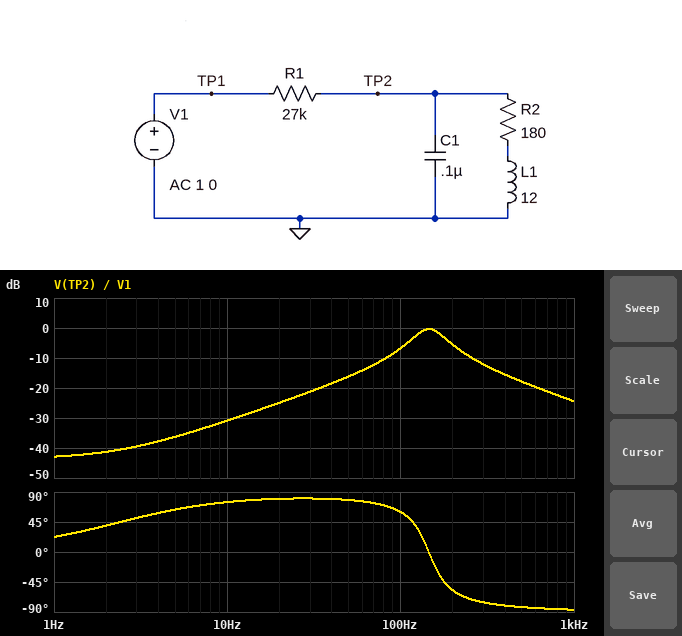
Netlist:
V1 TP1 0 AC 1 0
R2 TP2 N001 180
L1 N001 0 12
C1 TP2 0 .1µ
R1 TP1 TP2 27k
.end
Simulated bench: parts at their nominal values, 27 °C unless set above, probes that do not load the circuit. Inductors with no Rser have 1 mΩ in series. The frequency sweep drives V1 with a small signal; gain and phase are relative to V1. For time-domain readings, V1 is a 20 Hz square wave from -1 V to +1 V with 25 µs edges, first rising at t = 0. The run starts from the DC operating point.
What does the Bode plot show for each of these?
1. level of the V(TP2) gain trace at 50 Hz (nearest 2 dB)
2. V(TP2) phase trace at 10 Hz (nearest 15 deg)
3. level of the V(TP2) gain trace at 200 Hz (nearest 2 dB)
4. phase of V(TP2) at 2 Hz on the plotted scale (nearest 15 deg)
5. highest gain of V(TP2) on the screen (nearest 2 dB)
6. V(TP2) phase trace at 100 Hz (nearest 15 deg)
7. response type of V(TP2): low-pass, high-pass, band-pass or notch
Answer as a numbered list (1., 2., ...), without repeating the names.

1. -16 dB
2. 75 deg
3. -6 dB
4. 45 deg
5. 0 dB
6. 60 deg
7. band-pass
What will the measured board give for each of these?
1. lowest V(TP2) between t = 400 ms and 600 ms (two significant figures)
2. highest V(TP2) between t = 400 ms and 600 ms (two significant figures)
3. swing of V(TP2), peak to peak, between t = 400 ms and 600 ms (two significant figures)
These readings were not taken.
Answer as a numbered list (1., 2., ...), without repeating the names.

1. -610 mV
2. 610 mV
3. 1.2 V
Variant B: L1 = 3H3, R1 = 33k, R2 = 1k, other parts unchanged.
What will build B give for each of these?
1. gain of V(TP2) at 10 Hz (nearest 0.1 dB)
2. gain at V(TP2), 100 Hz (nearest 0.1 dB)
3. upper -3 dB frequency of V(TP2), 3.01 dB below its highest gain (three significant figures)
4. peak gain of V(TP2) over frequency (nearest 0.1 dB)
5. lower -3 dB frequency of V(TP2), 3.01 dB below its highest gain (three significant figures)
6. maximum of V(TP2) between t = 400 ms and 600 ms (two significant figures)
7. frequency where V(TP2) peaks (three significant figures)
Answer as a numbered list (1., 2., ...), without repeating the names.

1. -30.4 dB
2. -22.3 dB
3. 333 Hz
4. -5.9 dB
5. 237 Hz
6. 290 mV
7. 281 Hz
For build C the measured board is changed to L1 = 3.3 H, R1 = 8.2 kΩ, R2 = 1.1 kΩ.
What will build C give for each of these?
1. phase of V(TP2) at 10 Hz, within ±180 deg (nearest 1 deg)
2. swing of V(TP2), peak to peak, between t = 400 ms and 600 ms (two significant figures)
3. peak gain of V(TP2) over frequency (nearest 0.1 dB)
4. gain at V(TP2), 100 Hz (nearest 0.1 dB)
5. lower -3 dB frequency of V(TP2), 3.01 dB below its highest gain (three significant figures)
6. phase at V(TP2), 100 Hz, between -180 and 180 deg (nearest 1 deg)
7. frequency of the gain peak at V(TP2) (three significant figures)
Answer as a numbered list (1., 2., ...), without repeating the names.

1. 9 deg
2. 1.6 V
3. -2.0 dB
4. -11.3 dB
5. 193 Hz
6. 44 deg
7. 293 Hz
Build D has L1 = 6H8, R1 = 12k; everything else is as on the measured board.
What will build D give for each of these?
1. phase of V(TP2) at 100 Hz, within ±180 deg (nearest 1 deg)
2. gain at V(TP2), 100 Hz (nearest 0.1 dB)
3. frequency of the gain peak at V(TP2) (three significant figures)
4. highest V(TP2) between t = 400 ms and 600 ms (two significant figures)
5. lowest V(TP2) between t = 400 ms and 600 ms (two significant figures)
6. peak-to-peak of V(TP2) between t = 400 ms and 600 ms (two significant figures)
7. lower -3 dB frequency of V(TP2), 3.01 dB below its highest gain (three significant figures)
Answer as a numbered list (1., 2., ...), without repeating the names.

1. 61 deg
2. -7.4 dB
3. 194 Hz
4. 870 mV
5. -870 mV
6. 1.7 V
7. 138 Hz
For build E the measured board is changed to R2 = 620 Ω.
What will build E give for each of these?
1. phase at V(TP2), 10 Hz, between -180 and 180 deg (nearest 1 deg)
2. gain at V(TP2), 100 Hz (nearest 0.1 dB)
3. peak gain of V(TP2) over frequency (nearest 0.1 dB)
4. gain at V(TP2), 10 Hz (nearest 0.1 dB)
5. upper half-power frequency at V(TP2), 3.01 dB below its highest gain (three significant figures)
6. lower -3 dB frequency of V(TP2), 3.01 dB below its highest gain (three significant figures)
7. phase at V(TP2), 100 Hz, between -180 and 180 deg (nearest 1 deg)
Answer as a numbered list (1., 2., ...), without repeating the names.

1. 49 deg
2. -7.1 dB
3. -1.1 dB
4. -29.0 dB
5. 184 Hz
6. 117 Hz
7. 55 deg
